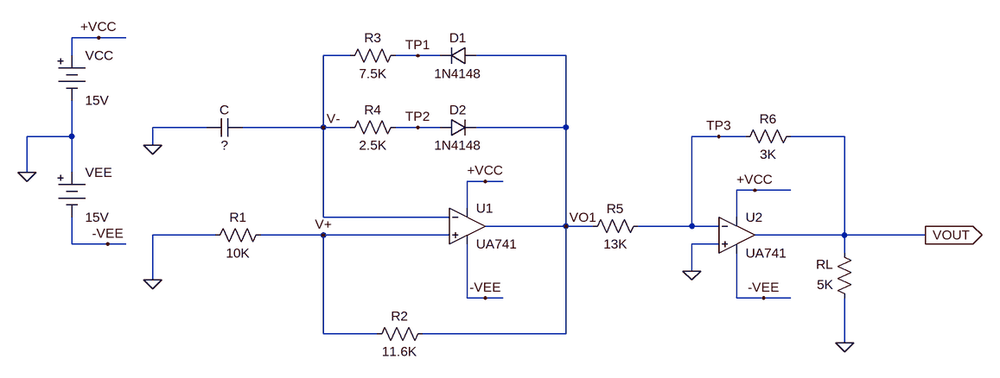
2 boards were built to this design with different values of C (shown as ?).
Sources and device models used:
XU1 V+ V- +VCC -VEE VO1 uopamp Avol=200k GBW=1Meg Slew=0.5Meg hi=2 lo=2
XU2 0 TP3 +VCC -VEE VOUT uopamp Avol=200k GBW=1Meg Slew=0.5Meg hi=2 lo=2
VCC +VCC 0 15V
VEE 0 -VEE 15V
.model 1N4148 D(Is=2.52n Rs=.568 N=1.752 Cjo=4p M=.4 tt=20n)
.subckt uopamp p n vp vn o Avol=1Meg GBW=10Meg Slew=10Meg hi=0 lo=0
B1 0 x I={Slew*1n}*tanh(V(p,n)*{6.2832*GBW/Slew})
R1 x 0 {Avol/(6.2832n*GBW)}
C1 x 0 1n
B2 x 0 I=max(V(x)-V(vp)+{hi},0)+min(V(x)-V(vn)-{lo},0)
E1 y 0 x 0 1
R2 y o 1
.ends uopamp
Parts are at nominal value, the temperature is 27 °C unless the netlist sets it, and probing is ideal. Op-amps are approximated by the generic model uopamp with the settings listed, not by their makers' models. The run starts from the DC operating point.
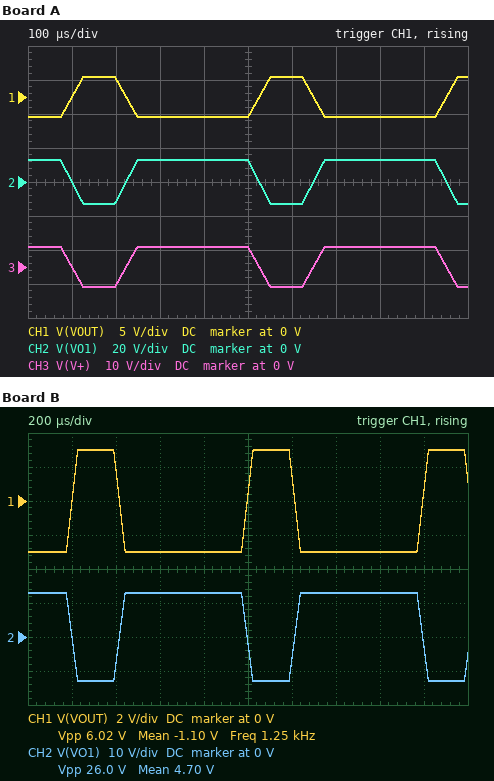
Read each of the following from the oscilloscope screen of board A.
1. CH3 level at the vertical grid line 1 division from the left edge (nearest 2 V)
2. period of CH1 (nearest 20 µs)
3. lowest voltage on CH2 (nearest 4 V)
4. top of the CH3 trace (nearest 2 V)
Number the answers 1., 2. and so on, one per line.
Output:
1. 0 V
2. 420 µs
3. -12 V
4. 6 V
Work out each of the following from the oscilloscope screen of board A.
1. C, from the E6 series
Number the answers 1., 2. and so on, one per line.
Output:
1. 33 nF
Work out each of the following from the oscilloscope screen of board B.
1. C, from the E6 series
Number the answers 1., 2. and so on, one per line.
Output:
1. 68 nF
